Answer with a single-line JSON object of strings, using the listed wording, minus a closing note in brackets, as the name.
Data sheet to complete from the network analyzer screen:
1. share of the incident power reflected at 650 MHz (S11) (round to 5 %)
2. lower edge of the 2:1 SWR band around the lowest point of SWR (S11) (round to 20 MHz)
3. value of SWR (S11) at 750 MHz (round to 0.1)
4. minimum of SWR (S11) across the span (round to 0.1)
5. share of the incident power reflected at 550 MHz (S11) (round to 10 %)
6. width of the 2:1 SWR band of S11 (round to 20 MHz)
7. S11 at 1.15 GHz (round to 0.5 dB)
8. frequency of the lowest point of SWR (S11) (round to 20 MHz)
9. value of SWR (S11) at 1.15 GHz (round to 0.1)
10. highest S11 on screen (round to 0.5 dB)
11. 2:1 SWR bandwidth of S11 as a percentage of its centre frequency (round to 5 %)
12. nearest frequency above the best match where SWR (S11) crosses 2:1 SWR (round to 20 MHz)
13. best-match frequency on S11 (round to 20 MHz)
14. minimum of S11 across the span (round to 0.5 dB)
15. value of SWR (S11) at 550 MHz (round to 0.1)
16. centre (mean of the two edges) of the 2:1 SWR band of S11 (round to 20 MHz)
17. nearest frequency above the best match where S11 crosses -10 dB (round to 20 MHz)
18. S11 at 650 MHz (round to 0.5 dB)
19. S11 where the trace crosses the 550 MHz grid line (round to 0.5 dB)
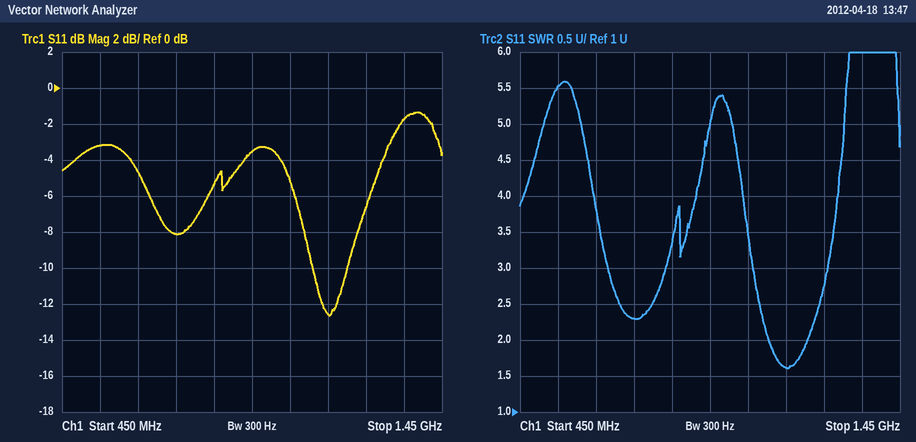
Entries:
{"share of the incident power reflected at 650 MHz (S11)": "35 %", "lower edge of the 2:1 SWR band around the lowest point of SWR (S11)": "1.10 GHz", "value of SWR (S11) at 750 MHz": "2.3", "minimum of SWR (S11) across the span": "1.6", "share of the incident power reflected at 550 MHz (S11)": "50 %", "width of the 2:1 SWR band of S11": "100 MHz", "S11 at 1.15 GHz": "-12.5 dB", "frequency of the lowest point of SWR (S11)": "1.16 GHz", "value of SWR (S11) at 1.15 GHz": "1.6", "highest S11 on screen": "-1.5 dB", "2:1 SWR bandwidth of S11 as a percentage of its centre frequency": "10 %", "nearest frequency above the best match where SWR (S11) crosses 2:1 SWR": "1.20 GHz", "best-match frequency on S11": "1.16 GHz", "minimum of S11 across the span": "-12.5 dB", "value of SWR (S11) at 550 MHz": "5.5", "centre (mean of the two edges) of the 2:1 SWR band of S11": "1.16 GHz", "nearest frequency above the best match where S11 crosses -10 dB": "1.20 GHz", "S11 at 650 MHz": "-4.5 dB", "S11 where the trace crosses the 550 MHz grid line": "-3.0 dB"}
